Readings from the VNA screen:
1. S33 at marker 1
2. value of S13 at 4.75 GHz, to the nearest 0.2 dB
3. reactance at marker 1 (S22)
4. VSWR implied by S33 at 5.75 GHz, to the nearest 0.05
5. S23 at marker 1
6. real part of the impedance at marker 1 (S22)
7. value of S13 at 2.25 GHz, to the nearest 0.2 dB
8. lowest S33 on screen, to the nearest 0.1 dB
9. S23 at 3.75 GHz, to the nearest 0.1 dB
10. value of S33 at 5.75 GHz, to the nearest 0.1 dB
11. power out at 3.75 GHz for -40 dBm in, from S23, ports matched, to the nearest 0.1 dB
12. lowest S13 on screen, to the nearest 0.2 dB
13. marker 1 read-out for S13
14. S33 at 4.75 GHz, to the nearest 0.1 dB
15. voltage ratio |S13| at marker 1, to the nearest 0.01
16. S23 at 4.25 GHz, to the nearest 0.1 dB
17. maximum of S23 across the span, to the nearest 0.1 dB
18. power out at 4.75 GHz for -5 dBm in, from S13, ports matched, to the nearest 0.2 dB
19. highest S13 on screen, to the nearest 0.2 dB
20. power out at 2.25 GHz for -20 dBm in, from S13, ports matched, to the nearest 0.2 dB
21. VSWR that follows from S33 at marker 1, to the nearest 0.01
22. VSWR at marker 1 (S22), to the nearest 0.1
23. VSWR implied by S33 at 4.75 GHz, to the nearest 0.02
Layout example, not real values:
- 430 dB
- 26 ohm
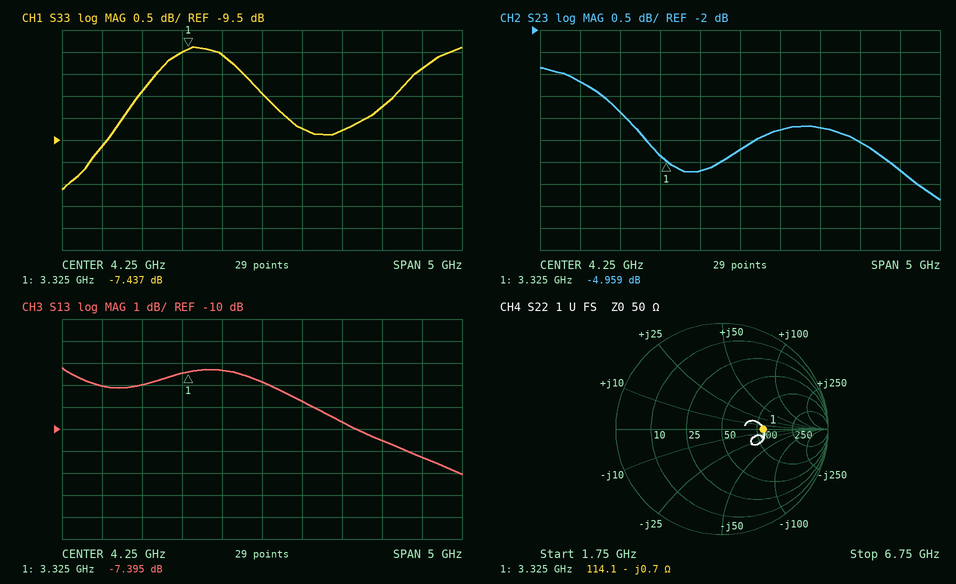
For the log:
- -7.437 dB
- -8.8 dB
- -0.7 Ω
- 2.15
- -4.959 dB
- 114.1 Ω
- -8.0 dB
- -10.6 dB
- -5.2 dB
- -8.7 dB
- -45.2 dBm
- -12.0 dB
- -7.395 dB
- -9.2 dB
- 0.43
- -4.7 dB
- -2.9 dB
- -13.8 dBm
- -7.2 dB
- -28.0 dBm
- 2.48
- 2.3
- 2.06
